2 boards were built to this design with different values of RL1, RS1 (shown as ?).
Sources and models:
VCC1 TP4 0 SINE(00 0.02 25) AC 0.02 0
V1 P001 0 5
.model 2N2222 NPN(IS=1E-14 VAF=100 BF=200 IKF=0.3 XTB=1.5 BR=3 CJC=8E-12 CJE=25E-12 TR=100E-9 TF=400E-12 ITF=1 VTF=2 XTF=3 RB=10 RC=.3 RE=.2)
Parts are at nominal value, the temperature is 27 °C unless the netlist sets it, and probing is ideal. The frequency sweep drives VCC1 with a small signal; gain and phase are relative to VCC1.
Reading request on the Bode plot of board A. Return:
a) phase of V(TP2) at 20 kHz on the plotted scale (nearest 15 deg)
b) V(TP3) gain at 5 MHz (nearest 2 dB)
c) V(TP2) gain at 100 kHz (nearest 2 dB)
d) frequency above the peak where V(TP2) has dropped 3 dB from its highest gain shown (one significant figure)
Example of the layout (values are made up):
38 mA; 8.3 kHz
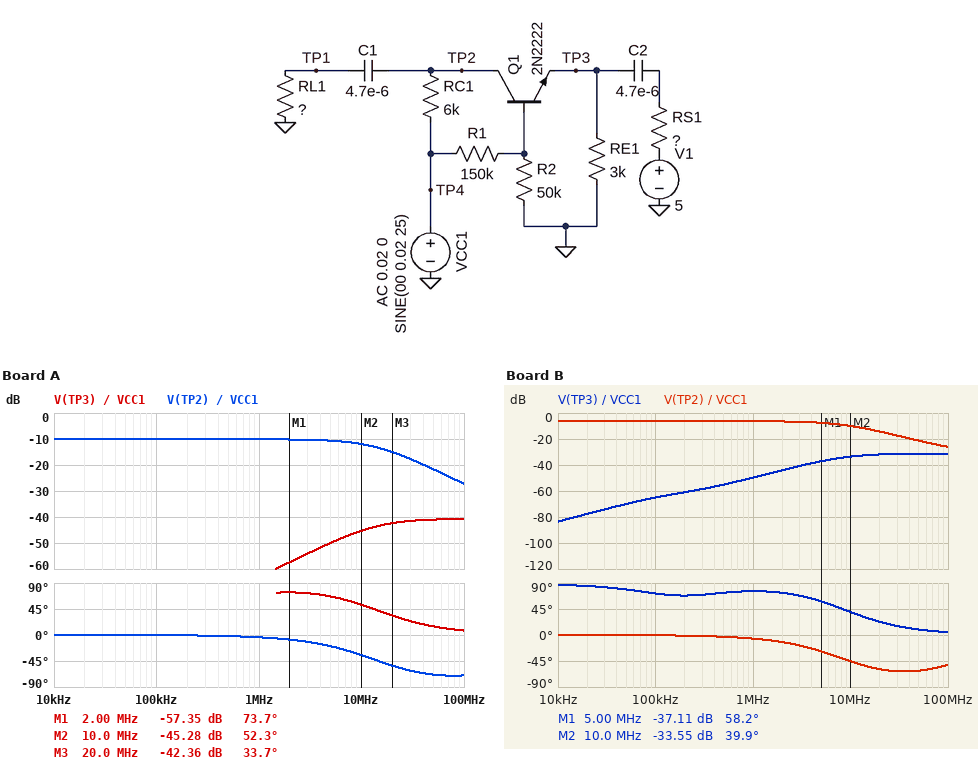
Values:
0 deg; -50 dB; -10 dB; 10 MHz
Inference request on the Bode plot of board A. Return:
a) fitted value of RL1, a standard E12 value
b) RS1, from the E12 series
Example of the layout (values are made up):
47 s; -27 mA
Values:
2.7 kΩ; 56 Ω
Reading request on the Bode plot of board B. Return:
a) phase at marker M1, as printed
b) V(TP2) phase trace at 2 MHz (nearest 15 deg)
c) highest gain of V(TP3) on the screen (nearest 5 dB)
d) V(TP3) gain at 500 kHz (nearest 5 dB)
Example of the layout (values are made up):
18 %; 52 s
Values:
58.2 deg; -15 deg; -30 dB; -55 dB
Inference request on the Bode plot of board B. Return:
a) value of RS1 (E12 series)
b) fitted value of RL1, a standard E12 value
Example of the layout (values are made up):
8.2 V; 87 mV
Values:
180 Ω; 5.6 kΩ
